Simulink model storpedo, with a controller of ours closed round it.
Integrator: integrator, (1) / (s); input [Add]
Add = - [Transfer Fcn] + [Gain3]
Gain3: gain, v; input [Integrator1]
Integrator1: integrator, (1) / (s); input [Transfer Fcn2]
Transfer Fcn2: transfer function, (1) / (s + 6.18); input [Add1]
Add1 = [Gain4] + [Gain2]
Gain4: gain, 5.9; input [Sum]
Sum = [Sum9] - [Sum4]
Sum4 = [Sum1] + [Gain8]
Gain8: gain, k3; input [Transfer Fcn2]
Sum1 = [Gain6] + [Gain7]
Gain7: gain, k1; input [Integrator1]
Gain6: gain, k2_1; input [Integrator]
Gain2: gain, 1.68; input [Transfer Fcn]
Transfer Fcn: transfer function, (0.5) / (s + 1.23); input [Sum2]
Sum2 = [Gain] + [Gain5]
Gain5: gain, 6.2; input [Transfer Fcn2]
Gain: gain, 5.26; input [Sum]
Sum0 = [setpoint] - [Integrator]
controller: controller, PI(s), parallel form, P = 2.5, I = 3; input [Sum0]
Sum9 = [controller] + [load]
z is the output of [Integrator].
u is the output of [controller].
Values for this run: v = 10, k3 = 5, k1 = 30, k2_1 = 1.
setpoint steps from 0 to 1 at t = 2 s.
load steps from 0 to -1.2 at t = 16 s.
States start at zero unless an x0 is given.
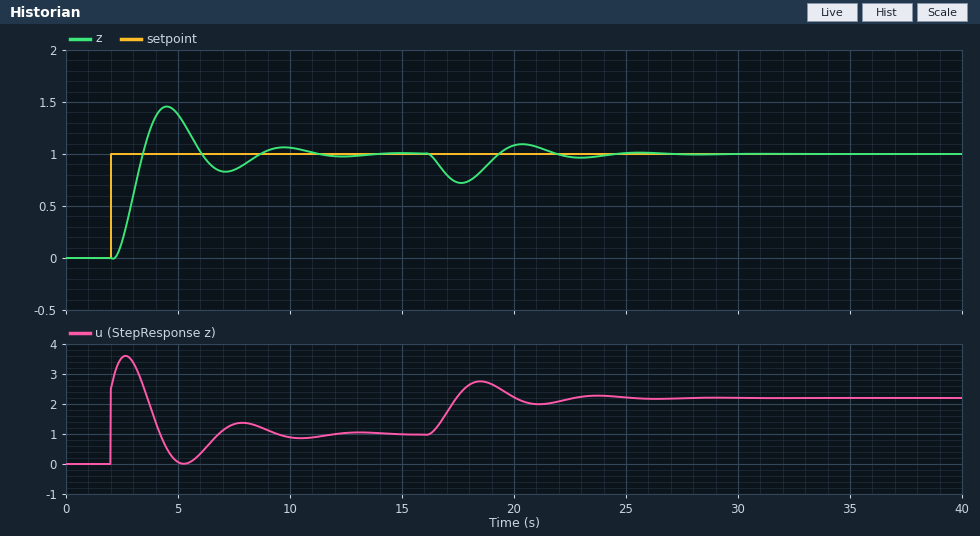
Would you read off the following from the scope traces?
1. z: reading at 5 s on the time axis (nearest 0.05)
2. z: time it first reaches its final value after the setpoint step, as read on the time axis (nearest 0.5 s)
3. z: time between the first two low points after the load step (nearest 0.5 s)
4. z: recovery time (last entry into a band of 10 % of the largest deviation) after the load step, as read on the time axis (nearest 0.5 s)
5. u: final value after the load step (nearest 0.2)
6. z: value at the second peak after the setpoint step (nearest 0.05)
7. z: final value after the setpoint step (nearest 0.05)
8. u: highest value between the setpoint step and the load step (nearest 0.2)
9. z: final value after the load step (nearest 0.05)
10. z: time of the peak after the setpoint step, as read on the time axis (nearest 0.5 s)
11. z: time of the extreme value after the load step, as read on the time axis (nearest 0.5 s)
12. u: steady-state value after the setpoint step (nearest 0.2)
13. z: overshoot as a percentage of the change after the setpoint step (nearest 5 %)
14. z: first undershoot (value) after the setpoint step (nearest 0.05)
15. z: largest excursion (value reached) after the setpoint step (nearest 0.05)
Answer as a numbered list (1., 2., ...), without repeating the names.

1. 1.40
2. 3.5 s
3. 5.5 s
4. 23.5 s
5. 2.2
6. 1.05
7. 1.00
8. 3.6
9. 1.00
10. 4.5 s
11. 17.5 s
12. 1.0
13. 45 %
14. 0.85
15. 1.45
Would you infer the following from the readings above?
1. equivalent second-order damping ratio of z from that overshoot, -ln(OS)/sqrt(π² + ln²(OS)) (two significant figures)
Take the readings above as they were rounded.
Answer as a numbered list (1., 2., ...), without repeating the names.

1. 0.25
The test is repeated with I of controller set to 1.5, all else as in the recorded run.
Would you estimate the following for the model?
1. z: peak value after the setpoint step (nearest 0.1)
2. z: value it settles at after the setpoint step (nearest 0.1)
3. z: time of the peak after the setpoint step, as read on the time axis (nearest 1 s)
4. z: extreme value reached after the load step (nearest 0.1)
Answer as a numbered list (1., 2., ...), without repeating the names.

1. 1.2
2. 1.0
3. 5 s
4. 0.7
